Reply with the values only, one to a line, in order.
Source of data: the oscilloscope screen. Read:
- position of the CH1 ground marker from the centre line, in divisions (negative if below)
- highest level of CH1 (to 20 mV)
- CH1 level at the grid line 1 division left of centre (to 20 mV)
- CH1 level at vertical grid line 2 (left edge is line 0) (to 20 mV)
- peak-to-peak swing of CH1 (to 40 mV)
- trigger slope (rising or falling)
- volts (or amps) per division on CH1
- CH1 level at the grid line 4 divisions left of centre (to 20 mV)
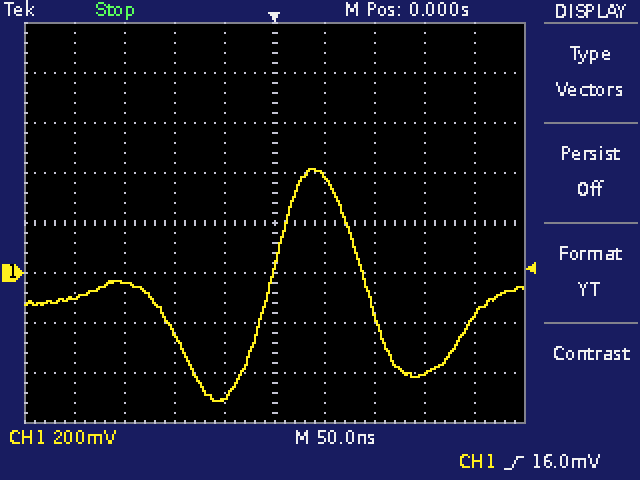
-1.0 div
420 mV
-500 mV
-40 mV
920 mV
rising
200 mV
-100 mV
